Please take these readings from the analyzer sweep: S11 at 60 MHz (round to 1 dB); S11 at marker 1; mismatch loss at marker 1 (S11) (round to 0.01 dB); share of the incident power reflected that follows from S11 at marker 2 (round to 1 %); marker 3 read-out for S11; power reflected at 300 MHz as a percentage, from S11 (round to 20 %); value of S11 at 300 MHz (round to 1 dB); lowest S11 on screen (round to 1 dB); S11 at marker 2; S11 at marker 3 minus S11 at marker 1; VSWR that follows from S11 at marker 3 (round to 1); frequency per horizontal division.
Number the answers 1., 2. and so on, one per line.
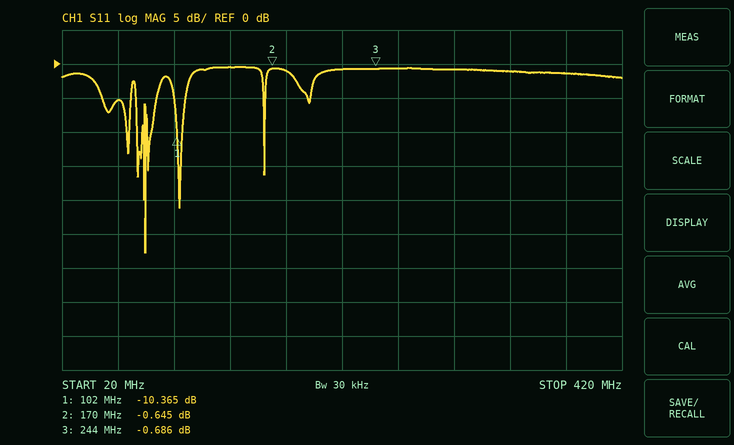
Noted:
1. -5 dB
2. -10.365 dB
3. 0.42 dB
4. 86 %
5. -0.686 dB
6. 80 %
7. -1 dB
8. -28 dB
9. -0.645 dB
10. 9.679 dB
11. 25
12. 40 MHz
